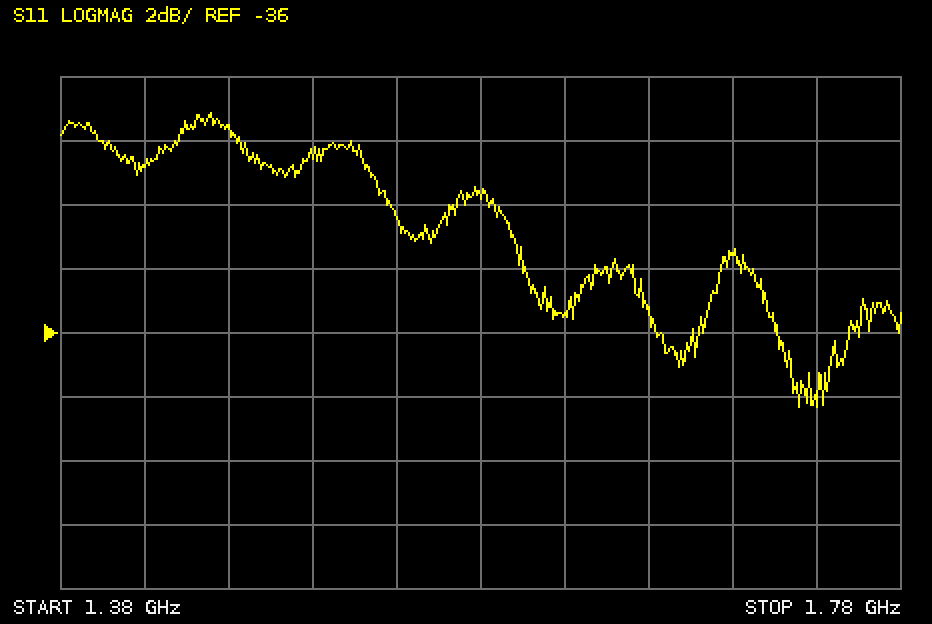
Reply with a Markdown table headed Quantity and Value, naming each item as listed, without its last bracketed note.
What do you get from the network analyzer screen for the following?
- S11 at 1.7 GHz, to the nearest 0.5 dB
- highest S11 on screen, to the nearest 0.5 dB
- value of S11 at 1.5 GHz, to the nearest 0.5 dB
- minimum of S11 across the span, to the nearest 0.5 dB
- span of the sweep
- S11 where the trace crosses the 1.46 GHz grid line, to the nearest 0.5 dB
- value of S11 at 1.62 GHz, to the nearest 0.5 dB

| Quantity | Value |
|---|---|
| S11 at 1.7 GHz, to the nearest 0.5 dB | -33.5 dB |
| highest S11 on screen, to the nearest 0.5 dB | -29.0 dB |
| value of S11 at 1.5 GHz, to the nearest 0.5 dB | -30.5 dB |
| minimum of S11 across the span, to the nearest 0.5 dB | -38.5 dB |
| span of the sweep | 400 MHz |
| S11 where the trace crosses the 1.46 GHz grid line, to the nearest 0.5 dB | -29.5 dB |
| value of S11 at 1.62 GHz, to the nearest 0.5 dB | -35.5 dB |
